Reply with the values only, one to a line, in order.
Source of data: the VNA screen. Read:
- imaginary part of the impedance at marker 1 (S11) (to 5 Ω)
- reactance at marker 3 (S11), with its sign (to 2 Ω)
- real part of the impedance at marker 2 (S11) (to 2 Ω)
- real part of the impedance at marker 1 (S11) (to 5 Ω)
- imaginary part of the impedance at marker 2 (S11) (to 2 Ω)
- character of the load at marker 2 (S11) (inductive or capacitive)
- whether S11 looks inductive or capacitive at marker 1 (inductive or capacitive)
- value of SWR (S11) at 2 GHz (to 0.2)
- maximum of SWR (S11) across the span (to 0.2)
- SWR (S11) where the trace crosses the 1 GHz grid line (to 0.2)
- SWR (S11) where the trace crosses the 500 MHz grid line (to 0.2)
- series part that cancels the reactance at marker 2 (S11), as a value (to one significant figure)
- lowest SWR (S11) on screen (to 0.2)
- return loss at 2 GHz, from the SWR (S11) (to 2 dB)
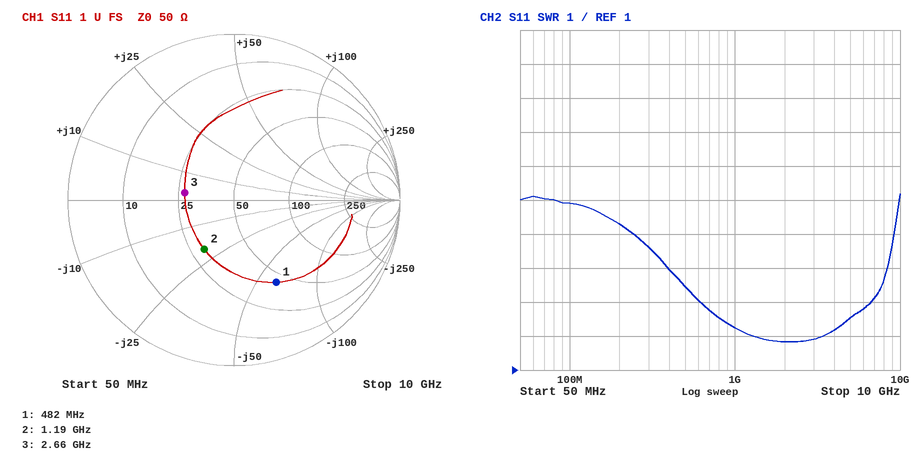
-60 Ω
+2 Ω
30 Ω
45 Ω
-20 Ω
capacitive
capacitive
1.8
6.2
2.2
3.4
3 nH
1.8
10 dB
